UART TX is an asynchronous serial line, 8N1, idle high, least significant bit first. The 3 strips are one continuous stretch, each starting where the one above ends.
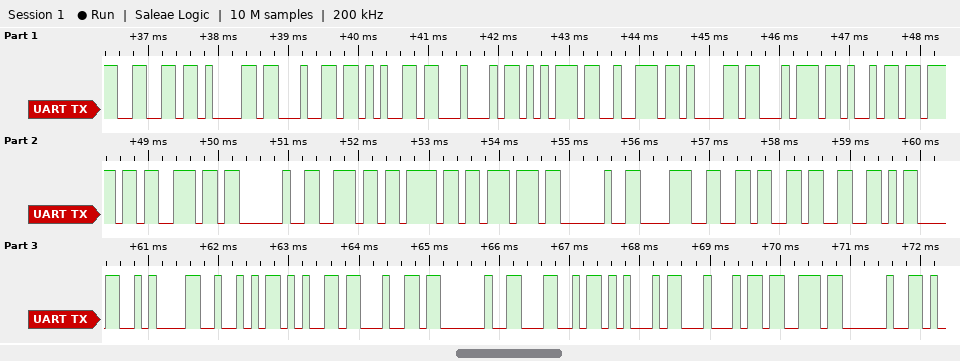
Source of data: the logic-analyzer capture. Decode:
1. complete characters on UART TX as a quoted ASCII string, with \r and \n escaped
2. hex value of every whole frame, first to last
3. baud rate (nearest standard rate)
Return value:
"fadeDuration now 863\r\nRed LEDs "
66 61 64 65 44 75 72 61 74 69 6F 6E 20 6E 6F 77 20 38 36 33 0D 0A 52 65 64 20 4C 45 44 73 20
9600 baud
